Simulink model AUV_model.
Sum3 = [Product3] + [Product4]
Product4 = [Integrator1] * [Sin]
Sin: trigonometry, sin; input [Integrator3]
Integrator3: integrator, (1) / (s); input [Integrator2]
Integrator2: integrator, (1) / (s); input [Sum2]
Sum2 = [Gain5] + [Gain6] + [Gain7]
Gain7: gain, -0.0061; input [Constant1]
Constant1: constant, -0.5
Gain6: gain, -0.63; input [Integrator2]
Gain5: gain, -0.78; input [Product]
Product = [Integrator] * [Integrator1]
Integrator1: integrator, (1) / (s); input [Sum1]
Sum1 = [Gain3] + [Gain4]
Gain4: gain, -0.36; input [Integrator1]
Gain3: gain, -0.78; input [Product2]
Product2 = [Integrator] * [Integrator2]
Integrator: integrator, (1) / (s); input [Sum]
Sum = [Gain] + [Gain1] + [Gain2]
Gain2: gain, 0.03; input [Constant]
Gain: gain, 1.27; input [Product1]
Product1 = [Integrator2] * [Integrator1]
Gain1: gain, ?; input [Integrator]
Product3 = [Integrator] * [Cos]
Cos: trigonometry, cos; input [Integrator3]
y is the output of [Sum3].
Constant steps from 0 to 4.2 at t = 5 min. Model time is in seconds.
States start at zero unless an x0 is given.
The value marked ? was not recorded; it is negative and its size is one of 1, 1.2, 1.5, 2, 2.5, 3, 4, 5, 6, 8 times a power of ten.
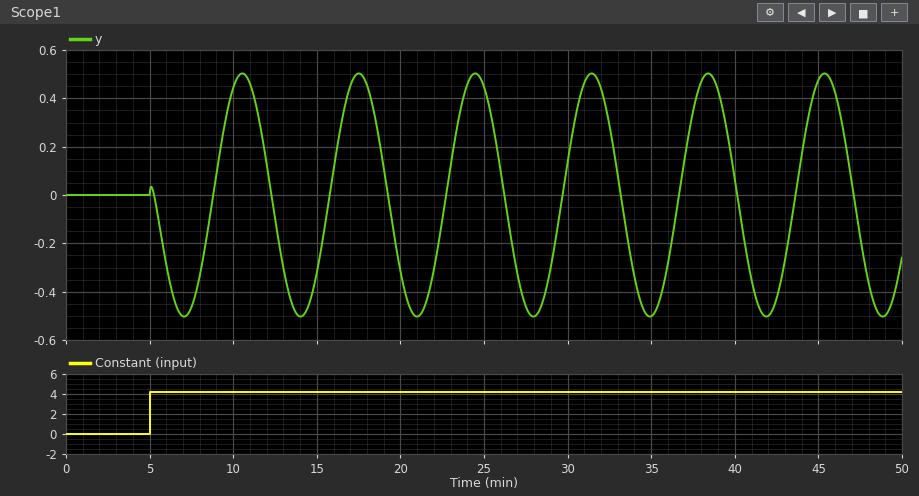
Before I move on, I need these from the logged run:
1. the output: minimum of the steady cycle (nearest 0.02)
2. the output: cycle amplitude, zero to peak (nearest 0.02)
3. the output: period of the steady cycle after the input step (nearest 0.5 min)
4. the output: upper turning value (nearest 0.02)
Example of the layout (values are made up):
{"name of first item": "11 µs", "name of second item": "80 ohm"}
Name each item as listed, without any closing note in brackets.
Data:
{"the output: minimum of the steady cycle": "-0.50", "the output: cycle amplitude, zero to peak": "0.50", "the output: period of the steady cycle after the input step": "7.0 min", "the output: upper turning value": "0.50"}
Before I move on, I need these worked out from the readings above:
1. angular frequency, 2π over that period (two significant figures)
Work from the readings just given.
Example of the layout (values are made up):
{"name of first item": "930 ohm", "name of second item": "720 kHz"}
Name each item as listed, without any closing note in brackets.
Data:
{"angular frequency, 2π over that period": "0.90 rad/min"}
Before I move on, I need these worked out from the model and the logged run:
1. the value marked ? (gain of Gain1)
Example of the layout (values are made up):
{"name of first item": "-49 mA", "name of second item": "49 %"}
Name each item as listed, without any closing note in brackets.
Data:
{"the value marked ?": "-0.25"}
